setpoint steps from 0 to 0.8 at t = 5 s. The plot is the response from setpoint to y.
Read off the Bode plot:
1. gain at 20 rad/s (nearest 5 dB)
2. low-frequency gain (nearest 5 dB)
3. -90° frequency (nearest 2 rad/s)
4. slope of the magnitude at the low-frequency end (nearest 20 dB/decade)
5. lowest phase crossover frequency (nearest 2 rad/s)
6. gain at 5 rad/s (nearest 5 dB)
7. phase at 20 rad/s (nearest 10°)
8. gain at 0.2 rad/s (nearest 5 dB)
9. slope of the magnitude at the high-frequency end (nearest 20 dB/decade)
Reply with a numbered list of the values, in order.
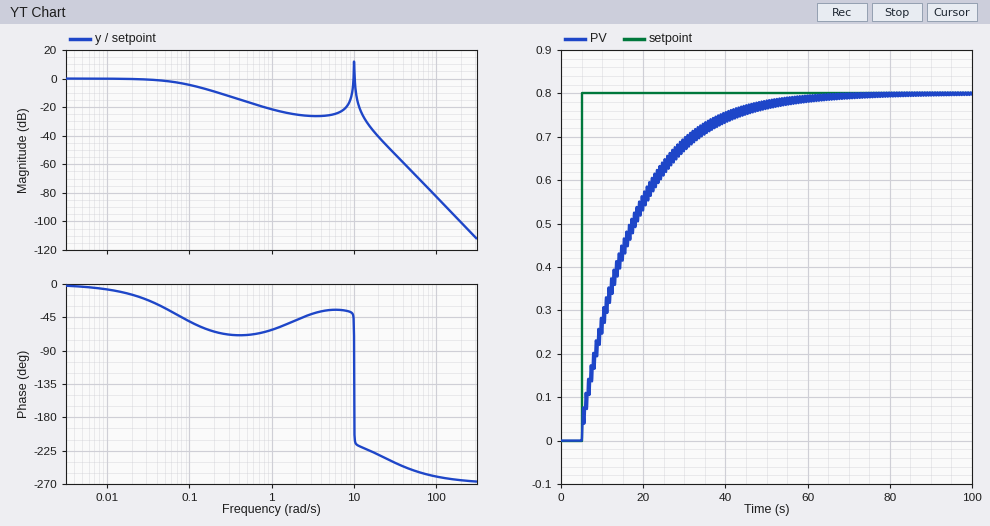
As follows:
1. -40 dB
2. 0 dB
3. 10 rad/s
4. 0 dB/decade
5. 10 rad/s
6. -25 dB
7. -230°
8. -10 dB
9. -60 dB/decade
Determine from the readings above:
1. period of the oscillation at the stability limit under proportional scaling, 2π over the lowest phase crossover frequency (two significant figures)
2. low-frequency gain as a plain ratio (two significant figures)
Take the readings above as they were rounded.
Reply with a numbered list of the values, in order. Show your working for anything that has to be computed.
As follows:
1. 2π / 10 = 0.63 s
2. 10^(0 / 20) = 1.0
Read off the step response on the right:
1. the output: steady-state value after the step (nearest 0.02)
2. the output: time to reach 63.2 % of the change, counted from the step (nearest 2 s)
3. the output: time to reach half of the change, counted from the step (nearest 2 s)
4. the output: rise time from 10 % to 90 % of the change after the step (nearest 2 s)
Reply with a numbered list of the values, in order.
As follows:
1. 0.80
2. 12 s
3. 8 s
4. 28 s
